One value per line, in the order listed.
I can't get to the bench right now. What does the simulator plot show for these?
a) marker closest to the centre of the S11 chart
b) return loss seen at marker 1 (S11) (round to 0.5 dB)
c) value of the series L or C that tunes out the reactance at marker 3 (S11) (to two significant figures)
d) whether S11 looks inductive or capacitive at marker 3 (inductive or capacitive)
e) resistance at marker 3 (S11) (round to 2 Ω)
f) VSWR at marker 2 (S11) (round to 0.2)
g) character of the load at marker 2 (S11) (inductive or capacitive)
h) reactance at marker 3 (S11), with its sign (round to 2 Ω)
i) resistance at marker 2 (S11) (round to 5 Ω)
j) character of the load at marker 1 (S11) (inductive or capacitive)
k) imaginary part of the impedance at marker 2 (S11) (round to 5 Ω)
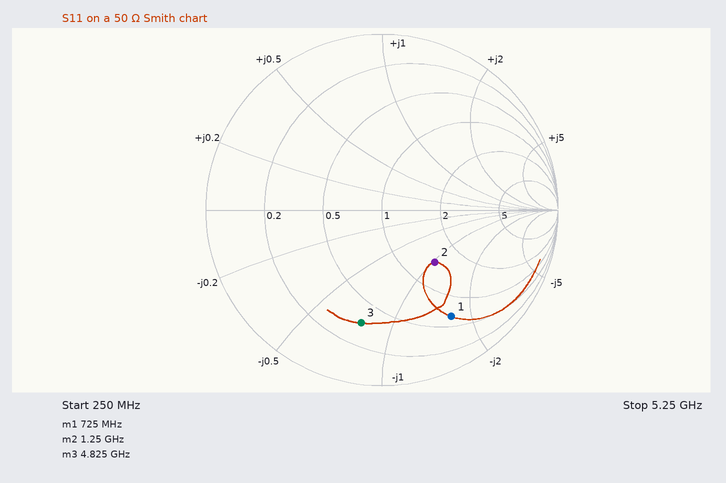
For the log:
marker 2
3.0 dB
1.3 nH
capacitive
18 Ω
2.4
capacitive
-38 Ω
70 Ω
capacitive
-50 Ω
